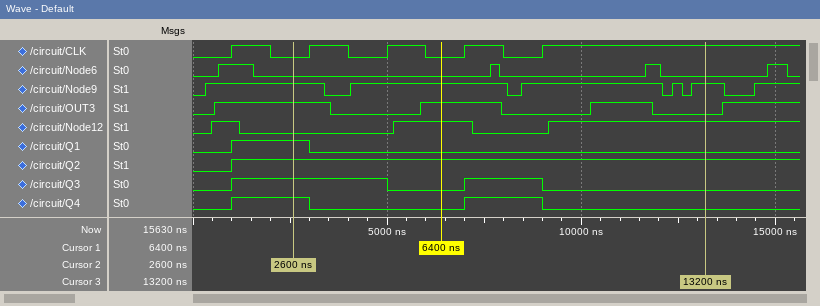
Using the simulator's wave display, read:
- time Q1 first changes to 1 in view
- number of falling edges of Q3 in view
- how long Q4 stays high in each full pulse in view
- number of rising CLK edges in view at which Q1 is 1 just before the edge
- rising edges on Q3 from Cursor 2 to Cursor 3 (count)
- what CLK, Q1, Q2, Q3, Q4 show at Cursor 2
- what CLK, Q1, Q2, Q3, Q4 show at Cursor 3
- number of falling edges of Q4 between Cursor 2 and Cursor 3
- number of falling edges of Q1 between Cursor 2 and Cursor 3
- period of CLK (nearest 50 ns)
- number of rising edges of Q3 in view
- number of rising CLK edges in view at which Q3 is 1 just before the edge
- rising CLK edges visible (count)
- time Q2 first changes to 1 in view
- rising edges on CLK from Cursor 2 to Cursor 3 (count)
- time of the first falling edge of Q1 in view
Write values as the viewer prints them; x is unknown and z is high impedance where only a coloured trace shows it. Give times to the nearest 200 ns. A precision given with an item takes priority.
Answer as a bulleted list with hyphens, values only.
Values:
- 1000 ns
- 2
- 2000 ns, 2000 ns
- 1
- 1
- CLK=0, Q1=1, Q2=1, Q3=1, Q4=1
- CLK=1, Q1=0, Q2=1, Q3=0, Q4=0
- 2
- 1
- 2000 ns
- 2
- 3
- 5
- 1000 ns
- 4
- 3000 ns
